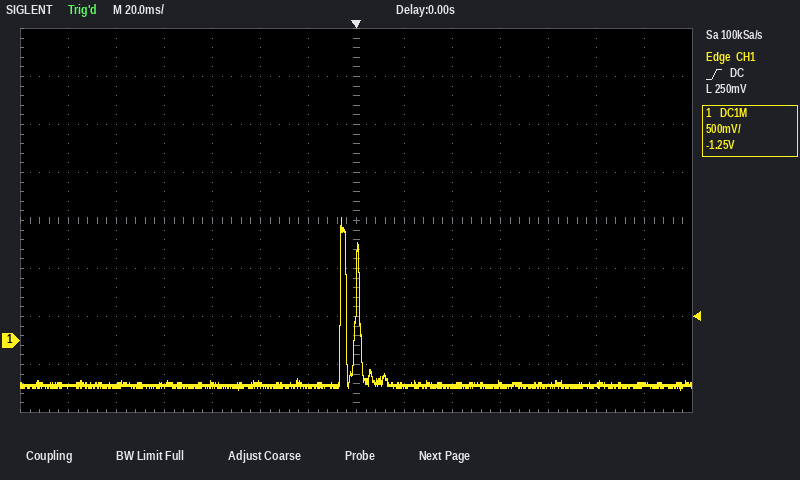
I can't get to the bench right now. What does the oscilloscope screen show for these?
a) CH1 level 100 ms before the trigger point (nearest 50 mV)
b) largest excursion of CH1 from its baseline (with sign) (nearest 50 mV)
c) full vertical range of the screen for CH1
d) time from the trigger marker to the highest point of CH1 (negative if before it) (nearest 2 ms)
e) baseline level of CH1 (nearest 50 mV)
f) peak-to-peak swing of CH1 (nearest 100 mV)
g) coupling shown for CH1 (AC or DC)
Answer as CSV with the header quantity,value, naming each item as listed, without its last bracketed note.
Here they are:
quantity,value
CH1 level 100 ms before the trigger point,-450 mV
largest excursion of CH1 from its baseline (with sign),+1.75 V
full vertical range of the screen for CH1,4 V
time from the trigger marker to the highest point of CH1 (negative if before it),-6 ms
baseline level of CH1,-450 mV
peak-to-peak swing of CH1,1.80 V
coupling shown for CH1,DC
